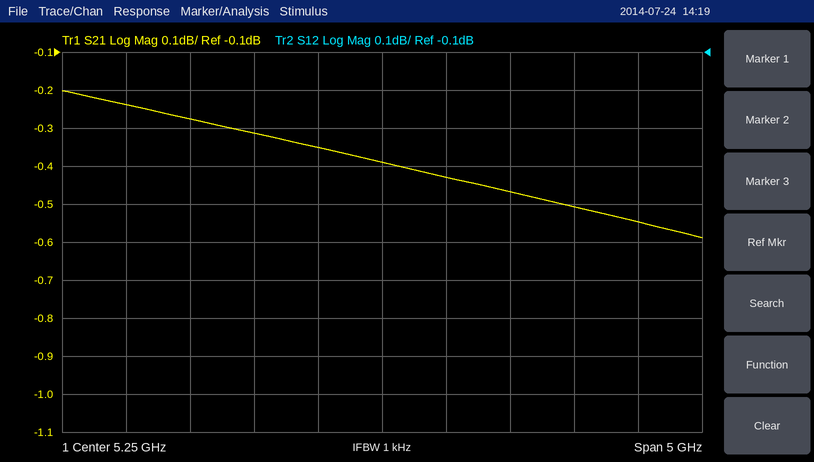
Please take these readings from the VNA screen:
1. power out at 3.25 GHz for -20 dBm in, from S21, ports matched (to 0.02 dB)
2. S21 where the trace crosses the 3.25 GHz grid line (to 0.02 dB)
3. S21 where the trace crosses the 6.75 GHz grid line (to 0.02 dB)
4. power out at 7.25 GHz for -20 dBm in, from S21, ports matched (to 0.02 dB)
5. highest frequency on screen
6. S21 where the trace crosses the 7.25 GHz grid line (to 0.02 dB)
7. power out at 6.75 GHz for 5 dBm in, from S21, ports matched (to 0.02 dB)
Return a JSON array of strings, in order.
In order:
["-20.24 dBm", "-0.24 dB", "-0.50 dB", "-20.54 dBm", "7.75 GHz", "-0.54 dB", "4.50 dBm"]
